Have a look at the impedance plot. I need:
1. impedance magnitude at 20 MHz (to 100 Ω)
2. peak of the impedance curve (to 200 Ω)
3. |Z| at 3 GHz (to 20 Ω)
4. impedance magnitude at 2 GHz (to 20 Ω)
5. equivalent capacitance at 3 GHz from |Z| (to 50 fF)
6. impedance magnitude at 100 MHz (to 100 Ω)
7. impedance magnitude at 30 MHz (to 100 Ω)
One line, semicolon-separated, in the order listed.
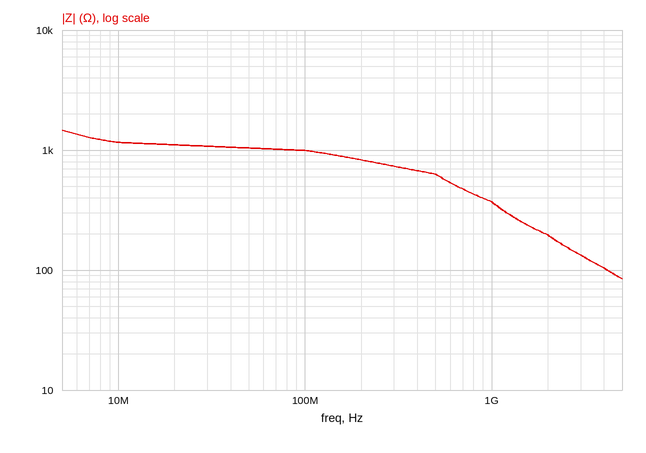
1.1 kΩ; 1.4 kΩ; 140 Ω; 200 Ω; 400 fF; 1.0 kΩ; 1.1 kΩ
